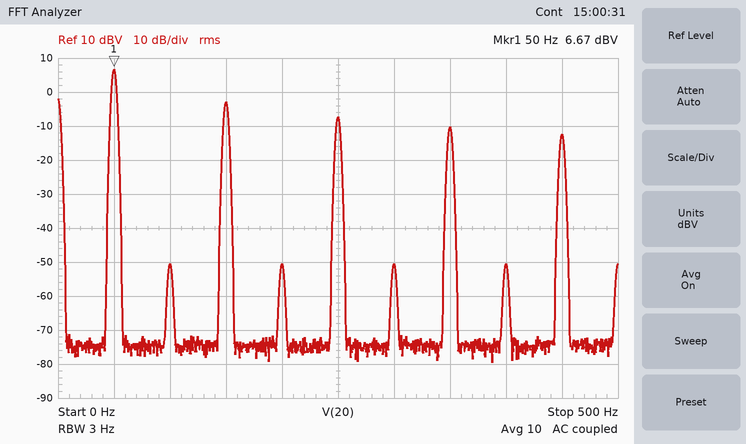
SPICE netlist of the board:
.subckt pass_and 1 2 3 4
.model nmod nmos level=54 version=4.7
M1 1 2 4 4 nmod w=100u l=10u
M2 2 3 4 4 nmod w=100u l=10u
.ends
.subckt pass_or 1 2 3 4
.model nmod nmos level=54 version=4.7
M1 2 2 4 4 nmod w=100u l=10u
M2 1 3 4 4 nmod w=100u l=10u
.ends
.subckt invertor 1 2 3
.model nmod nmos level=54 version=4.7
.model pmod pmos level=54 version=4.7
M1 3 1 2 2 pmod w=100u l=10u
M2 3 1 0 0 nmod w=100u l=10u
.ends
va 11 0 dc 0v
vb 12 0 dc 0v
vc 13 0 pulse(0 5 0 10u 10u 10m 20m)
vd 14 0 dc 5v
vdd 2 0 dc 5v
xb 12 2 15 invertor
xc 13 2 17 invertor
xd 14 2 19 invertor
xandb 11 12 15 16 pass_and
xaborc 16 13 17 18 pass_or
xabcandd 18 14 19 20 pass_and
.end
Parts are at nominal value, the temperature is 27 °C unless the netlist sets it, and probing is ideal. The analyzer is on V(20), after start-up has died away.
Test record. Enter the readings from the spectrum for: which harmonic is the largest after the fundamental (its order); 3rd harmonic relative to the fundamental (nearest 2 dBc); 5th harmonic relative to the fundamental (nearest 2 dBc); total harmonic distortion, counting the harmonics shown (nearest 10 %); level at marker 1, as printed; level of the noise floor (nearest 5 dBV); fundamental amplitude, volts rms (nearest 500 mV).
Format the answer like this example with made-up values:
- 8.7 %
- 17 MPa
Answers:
- 3
- -10 dBc
- -14 dBc
- 40 %
- 6.67 dBV
- -75 dBV
- 2.0 V
